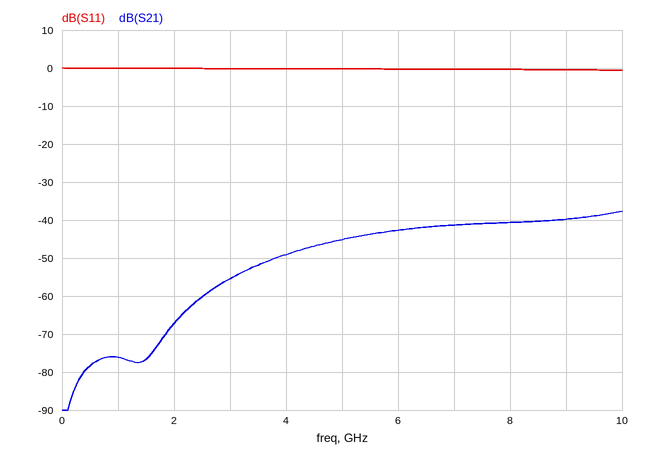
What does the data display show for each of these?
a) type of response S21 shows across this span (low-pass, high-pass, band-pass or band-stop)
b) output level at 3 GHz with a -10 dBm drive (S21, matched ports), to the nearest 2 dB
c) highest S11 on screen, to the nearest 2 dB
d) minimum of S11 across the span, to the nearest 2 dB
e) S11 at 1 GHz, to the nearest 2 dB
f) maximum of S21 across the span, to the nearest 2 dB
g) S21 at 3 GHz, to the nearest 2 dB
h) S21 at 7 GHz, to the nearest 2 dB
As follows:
high-pass
-66 dBm
0 dB
0 dB
0 dB
-38 dB
-56 dB
-42 dB
